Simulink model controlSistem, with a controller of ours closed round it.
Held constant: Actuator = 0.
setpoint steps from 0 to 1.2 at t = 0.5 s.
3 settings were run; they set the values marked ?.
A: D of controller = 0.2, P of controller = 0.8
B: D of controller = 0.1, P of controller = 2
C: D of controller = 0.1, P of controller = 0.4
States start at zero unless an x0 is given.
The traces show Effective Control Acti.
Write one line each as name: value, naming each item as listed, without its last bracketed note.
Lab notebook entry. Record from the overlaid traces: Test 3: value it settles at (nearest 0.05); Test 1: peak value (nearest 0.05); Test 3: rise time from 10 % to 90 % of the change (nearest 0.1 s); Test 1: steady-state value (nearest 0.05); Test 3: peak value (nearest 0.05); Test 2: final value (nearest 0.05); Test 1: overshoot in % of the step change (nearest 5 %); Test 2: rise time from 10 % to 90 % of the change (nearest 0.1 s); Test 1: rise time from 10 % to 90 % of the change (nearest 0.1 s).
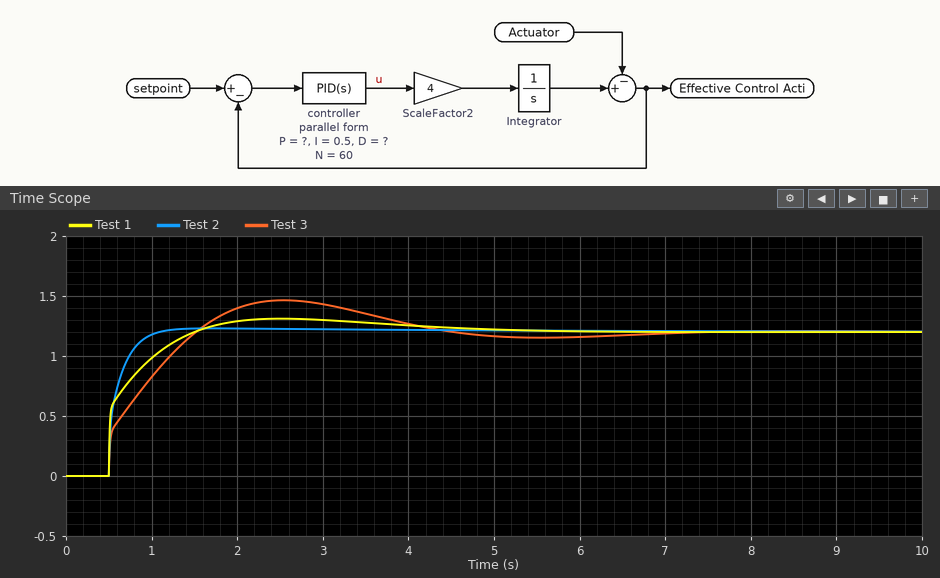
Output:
Test 3: value it settles at: 1.20
Test 1: peak value: 1.30
Test 3: rise time from 10 % to 90 % of the change: 0.8 s
Test 1: steady-state value: 1.20
Test 3: peak value: 1.45
Test 2: final value: 1.20
Test 1: overshoot in % of the step change: 10 %
Test 2: rise time from 10 % to 90 % of the change: 0.3 s
Test 1: rise time from 10 % to 90 % of the change: 0.7 s
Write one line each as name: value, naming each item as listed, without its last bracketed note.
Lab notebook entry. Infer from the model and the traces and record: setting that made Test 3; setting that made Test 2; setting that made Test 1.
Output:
setting that made Test 3: C
setting that made Test 2: B
setting that made Test 1: A
